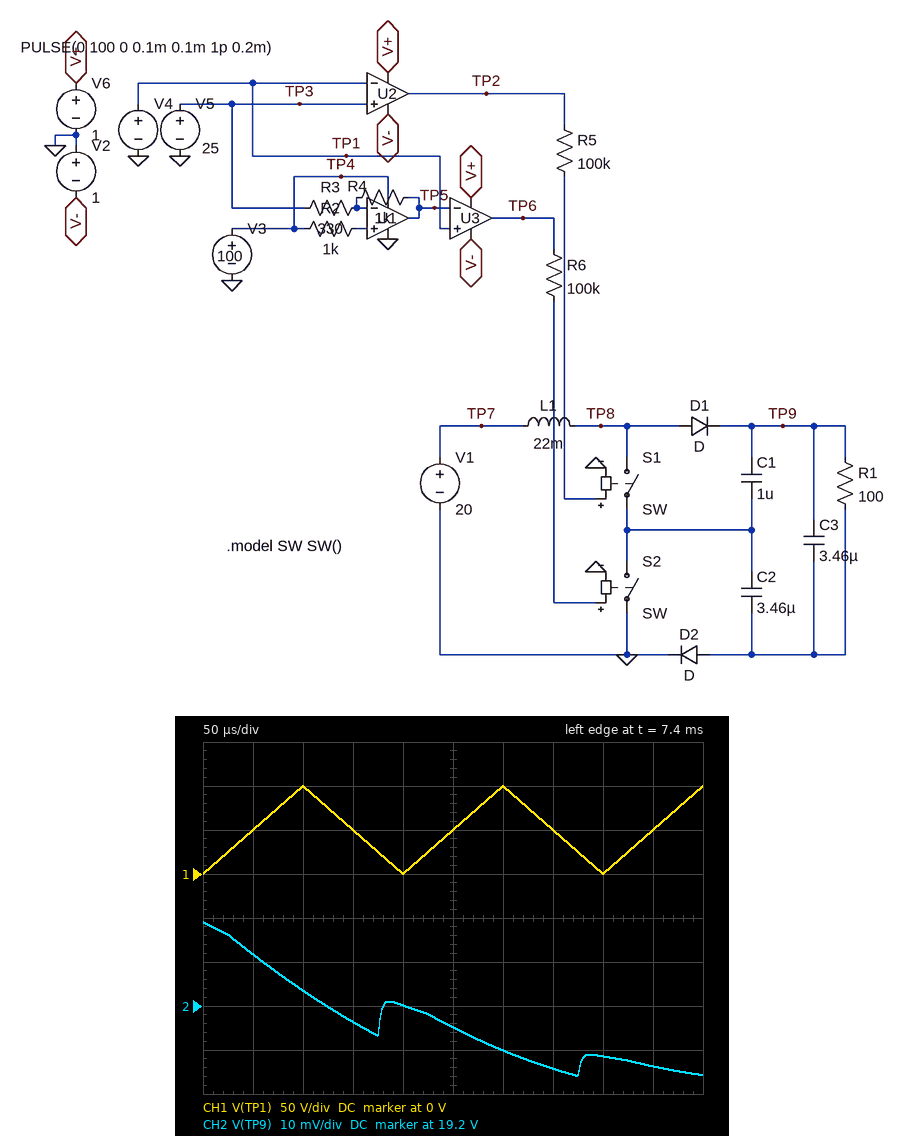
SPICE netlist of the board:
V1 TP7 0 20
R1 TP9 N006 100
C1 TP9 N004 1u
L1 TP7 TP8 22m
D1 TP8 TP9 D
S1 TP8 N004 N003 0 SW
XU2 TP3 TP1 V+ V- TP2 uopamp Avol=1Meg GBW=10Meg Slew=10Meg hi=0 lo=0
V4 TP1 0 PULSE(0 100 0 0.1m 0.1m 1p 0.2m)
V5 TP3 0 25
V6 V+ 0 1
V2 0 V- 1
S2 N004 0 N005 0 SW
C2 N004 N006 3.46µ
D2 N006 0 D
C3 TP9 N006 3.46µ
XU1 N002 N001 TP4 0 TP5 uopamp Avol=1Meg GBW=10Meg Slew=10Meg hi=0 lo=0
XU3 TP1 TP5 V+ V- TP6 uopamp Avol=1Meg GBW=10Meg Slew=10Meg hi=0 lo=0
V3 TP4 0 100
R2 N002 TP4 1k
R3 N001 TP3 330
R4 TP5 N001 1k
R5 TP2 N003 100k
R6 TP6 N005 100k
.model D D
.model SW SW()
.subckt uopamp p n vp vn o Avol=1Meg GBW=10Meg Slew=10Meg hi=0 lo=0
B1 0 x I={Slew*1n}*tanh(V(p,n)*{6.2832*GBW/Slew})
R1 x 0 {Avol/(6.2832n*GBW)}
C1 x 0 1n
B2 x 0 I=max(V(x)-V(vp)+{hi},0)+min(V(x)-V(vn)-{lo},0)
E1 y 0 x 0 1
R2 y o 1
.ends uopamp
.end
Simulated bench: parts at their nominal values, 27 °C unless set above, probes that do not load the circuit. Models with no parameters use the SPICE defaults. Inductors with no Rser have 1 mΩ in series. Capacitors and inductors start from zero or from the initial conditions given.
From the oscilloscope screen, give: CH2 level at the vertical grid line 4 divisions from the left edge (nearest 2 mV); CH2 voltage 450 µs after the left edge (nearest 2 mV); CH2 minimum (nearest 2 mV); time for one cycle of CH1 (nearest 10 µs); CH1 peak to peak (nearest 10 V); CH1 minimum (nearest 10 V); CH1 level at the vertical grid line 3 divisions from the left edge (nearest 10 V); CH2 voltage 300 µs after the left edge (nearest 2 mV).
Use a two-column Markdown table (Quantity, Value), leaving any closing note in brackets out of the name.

| Quantity | Value |
|---|---|
| CH2 level at the vertical grid line 4 divisions from the left edge | 19.200 V |
| CH2 voltage 450 µs after the left edge | 19.186 V |
| CH2 minimum | 19.184 V |
| time for one cycle of CH1 | 200 µs |
| CH1 peak to peak | 100 V |
| CH1 minimum | 0 V |
| CH1 level at the vertical grid line 3 divisions from the left edge | 50 V |
| CH2 voltage 300 µs after the left edge | 19.190 V |
